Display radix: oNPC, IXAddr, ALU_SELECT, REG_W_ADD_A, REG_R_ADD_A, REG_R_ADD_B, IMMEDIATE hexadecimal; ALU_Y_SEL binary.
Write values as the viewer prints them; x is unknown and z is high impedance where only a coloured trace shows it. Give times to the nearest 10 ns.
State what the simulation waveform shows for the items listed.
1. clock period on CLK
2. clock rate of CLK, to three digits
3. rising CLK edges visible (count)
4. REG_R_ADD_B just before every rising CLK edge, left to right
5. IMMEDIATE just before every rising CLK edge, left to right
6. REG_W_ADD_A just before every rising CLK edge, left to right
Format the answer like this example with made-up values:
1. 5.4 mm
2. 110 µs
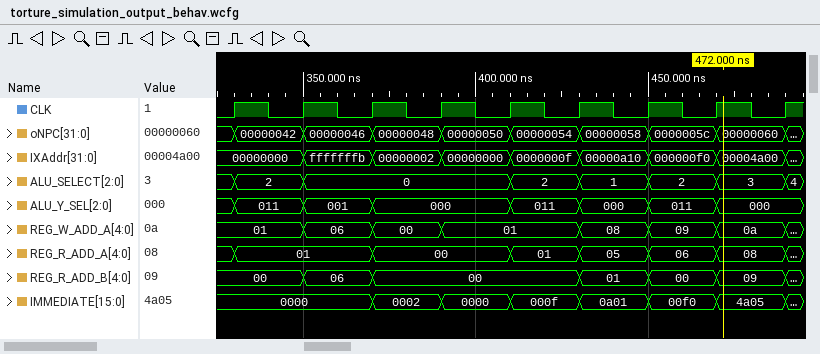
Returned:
1. 20 ns
2. 50.0 MHz
3. 9
4. 00, 00, 06, 00, 00, 00, 01, 00, 09
5. 0000, 0000, 0000, 0002, 0000, 000f, 0a01, 00f0, 4a05
6. 01, 01, 06, 00, 01, 01, 08, 09, 0a
